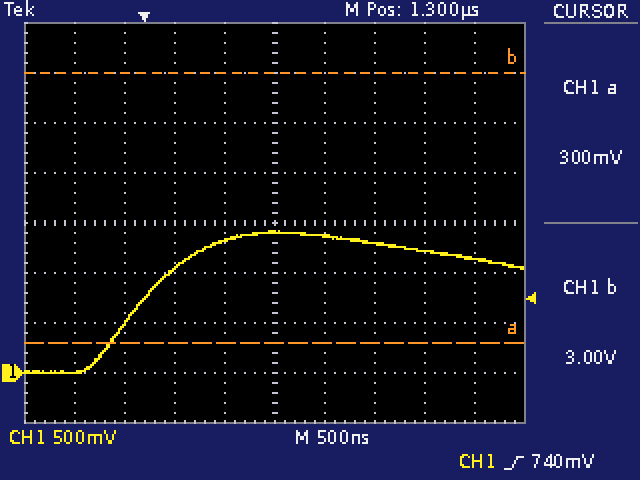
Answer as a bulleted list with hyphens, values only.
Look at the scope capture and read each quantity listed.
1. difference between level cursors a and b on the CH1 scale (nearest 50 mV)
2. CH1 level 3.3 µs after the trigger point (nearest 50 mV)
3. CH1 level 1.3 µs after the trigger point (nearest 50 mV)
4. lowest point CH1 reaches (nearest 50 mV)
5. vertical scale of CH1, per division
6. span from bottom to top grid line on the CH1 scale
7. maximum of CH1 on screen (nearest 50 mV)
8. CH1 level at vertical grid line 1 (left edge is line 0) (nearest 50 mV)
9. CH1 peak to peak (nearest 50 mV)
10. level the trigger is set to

- 2.70 V
- 1.15 V
- 1.40 V
- 0 mV
- 500 mV
- 4 V
- 1.40 V
- 0 mV
- 1.40 V
- 740 mV
